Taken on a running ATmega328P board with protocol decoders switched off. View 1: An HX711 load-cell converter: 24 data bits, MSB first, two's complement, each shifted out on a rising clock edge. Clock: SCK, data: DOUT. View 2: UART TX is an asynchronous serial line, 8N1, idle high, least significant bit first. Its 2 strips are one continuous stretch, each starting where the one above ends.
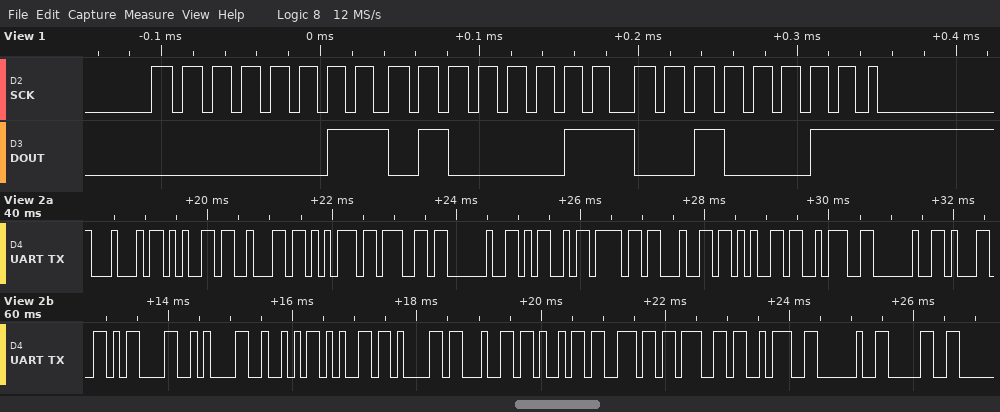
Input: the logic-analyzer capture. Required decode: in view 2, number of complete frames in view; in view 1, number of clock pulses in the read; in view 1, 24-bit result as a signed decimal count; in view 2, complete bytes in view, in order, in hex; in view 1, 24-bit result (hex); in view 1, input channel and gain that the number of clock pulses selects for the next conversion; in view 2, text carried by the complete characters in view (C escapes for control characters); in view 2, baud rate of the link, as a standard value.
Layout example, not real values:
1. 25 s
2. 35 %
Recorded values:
1. 25
2. 25
3. 213795
4. 0x44 0x65 0x62 0x75 0x67 0x20 0x4D 0x6F 0x64 0x65 0x3A 0x20 0x31 0x0D 0x0A 0x52 0x65 0x61 0x64 0x69 0x6E 0x67 0x3A 0x20 0x30
5. 0x034323
6. channel A, gain 128
7. "Debug Mode: 1\r\nReading: 0"
8. 9600 baud
